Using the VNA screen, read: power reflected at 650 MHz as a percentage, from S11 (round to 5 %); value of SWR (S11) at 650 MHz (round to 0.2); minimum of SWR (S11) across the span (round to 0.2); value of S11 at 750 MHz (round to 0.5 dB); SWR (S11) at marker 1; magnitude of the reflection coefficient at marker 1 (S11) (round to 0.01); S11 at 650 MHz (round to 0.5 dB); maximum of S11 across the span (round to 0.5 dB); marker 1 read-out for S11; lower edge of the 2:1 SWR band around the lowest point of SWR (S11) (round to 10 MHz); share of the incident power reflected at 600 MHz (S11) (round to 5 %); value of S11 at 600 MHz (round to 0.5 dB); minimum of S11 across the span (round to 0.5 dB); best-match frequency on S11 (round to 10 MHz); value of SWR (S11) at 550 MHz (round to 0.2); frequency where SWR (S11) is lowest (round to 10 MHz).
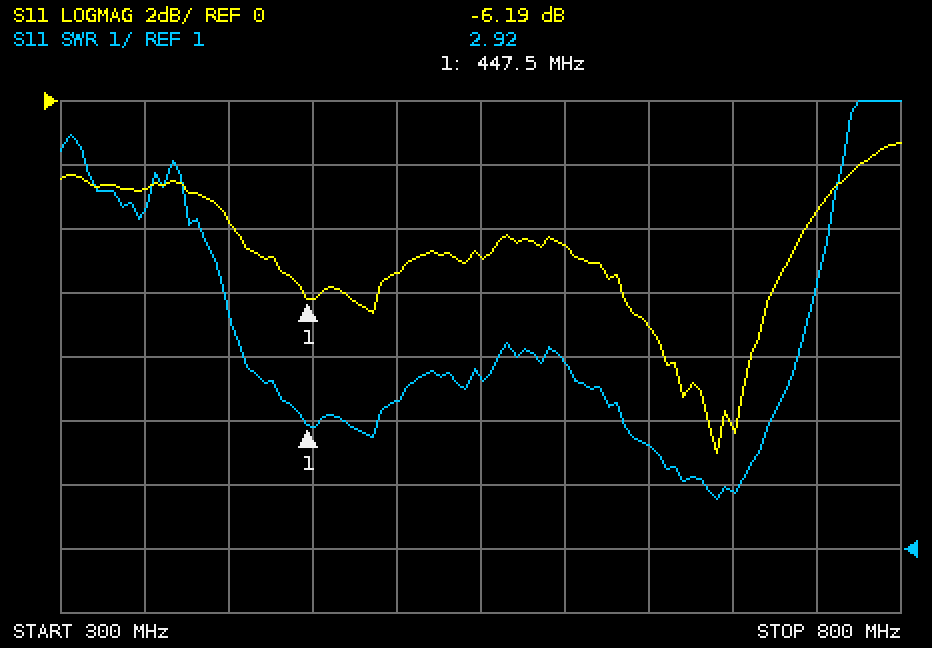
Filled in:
20 %
2.6
1.8
-3.5 dB
2.92
0.49
-7.0 dB
-1.5 dB
-6.19 dB
680 MHz
35 %
-4.5 dB
-11.0 dB
690 MHz
3.6
690 MHz
